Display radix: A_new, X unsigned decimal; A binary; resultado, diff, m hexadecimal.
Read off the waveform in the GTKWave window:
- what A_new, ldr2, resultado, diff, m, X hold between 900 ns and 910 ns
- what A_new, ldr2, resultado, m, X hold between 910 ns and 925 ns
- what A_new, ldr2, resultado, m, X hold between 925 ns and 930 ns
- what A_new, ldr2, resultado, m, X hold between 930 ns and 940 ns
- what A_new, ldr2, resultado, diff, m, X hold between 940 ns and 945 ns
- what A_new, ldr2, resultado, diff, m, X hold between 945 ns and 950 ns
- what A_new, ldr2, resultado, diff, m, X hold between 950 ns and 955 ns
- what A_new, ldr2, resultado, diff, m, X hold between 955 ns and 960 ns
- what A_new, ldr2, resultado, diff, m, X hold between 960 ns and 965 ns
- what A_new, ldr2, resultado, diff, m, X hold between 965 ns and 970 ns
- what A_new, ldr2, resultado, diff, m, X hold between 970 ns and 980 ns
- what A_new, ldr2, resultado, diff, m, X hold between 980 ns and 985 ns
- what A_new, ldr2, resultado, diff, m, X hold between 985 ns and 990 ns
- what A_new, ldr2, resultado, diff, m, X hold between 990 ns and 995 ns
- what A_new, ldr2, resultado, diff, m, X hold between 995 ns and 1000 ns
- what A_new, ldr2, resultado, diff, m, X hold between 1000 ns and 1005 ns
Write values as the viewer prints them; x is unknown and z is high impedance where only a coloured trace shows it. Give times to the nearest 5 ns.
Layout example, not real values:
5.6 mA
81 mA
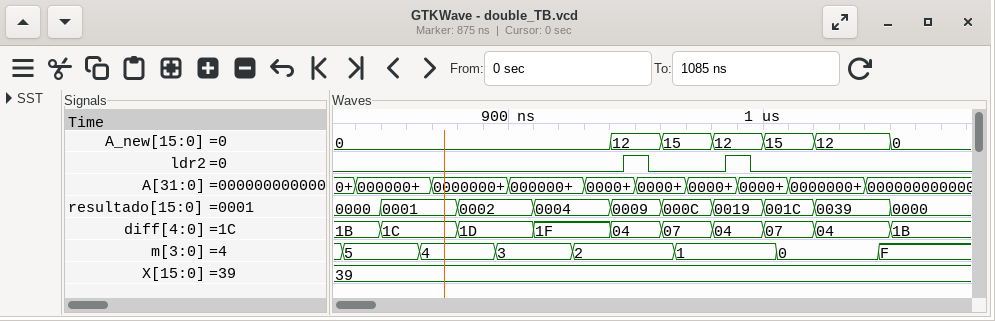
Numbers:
A_new=0, ldr2=0, resultado=0002, diff=1D, m=3, X=39
A_new=0, ldr2=0, resultado=0004, m=3, X=39
A_new=0, ldr2=0, resultado=0004, m=2, X=39
A_new=0, ldr2=0, resultado=0004, m=2, X=39
A_new=12, ldr2=0, resultado=0009, diff=04, m=2, X=39
A_new=12, ldr2=1, resultado=0009, diff=04, m=2, X=39
A_new=12, ldr2=1, resultado=0009, diff=04, m=2, X=39
A_new=12, ldr2=0, resultado=0009, diff=04, m=2, X=39
A_new=15, ldr2=0, resultado=000C, diff=07, m=2, X=39
A_new=15, ldr2=0, resultado=000C, diff=07, m=1, X=39
A_new=15, ldr2=0, resultado=000C, diff=07, m=1, X=39
A_new=12, ldr2=0, resultado=0019, diff=04, m=1, X=39
A_new=12, ldr2=1, resultado=0019, diff=04, m=1, X=39
A_new=12, ldr2=1, resultado=0019, diff=04, m=1, X=39
A_new=12, ldr2=0, resultado=0019, diff=04, m=1, X=39
A_new=15, ldr2=0, resultado=001C, diff=07, m=1, X=39
